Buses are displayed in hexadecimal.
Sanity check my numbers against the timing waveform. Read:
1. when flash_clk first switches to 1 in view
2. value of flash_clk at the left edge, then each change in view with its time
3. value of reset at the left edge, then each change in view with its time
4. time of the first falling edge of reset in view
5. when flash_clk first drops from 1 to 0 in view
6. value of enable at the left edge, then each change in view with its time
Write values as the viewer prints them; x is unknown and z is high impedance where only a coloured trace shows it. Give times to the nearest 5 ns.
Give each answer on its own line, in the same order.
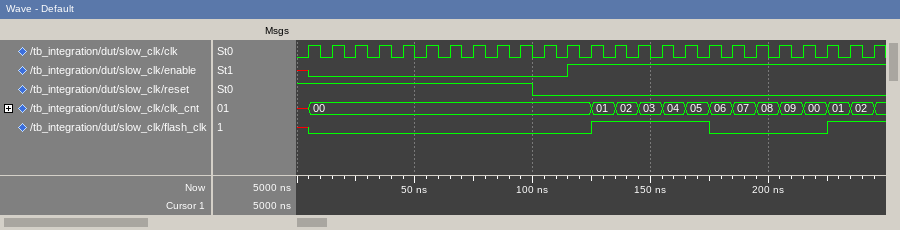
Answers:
125 ns
x, 0 at 5 ns, 1 at 125 ns, 0 at 175 ns, 1 at 225 ns
1, 0 at 100 ns
100 ns
175 ns
x, 0 at 5 ns, 1 at 115 ns
